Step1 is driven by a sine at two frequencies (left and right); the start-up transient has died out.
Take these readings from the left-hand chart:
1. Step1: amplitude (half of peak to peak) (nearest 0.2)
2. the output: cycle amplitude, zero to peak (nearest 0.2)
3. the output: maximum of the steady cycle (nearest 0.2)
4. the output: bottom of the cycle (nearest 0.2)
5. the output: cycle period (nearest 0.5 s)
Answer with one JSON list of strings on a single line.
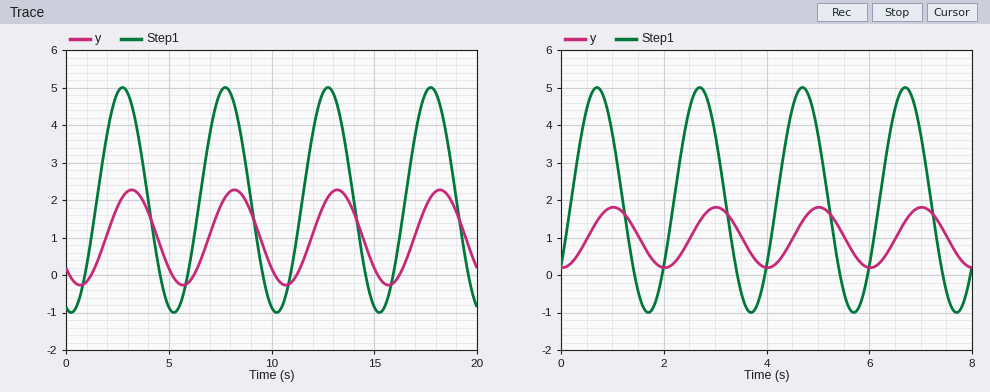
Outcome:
["3.0", "1.2", "2.2", "-0.2", "5.0 s"]
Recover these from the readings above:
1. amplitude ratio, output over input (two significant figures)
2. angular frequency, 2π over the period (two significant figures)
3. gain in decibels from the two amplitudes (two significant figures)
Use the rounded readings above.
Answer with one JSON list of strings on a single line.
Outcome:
["0.40", "1.3 rad/s", "-8.0 dB"]
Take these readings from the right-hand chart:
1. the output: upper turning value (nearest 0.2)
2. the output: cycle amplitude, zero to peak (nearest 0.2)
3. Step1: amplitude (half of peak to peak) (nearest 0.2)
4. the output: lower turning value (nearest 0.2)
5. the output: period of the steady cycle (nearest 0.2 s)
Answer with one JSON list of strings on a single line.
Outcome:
["1.8", "0.8", "3.0", "0.2", "2.0 s"]
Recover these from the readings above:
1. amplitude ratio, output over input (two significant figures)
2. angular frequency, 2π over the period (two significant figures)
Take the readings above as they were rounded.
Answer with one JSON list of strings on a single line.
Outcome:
["0.27", "3.1 rad/s"]
